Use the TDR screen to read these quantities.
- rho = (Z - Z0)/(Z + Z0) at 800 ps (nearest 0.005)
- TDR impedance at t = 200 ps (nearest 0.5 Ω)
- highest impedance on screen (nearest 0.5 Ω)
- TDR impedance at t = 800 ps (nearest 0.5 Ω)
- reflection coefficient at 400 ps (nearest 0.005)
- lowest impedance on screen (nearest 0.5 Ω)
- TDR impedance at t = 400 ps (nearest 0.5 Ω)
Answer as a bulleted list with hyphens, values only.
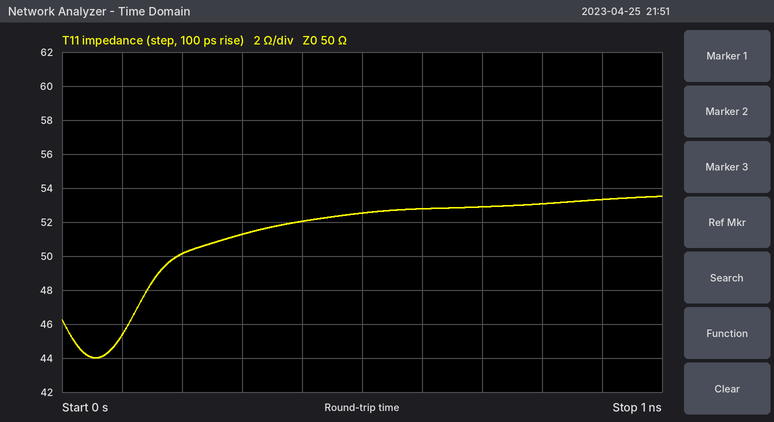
- +0.030
- 50.0 Ω
- 53.5 Ω
- 53.0 Ω
- +0.020
- 44.0 Ω
- 52.0 Ω
